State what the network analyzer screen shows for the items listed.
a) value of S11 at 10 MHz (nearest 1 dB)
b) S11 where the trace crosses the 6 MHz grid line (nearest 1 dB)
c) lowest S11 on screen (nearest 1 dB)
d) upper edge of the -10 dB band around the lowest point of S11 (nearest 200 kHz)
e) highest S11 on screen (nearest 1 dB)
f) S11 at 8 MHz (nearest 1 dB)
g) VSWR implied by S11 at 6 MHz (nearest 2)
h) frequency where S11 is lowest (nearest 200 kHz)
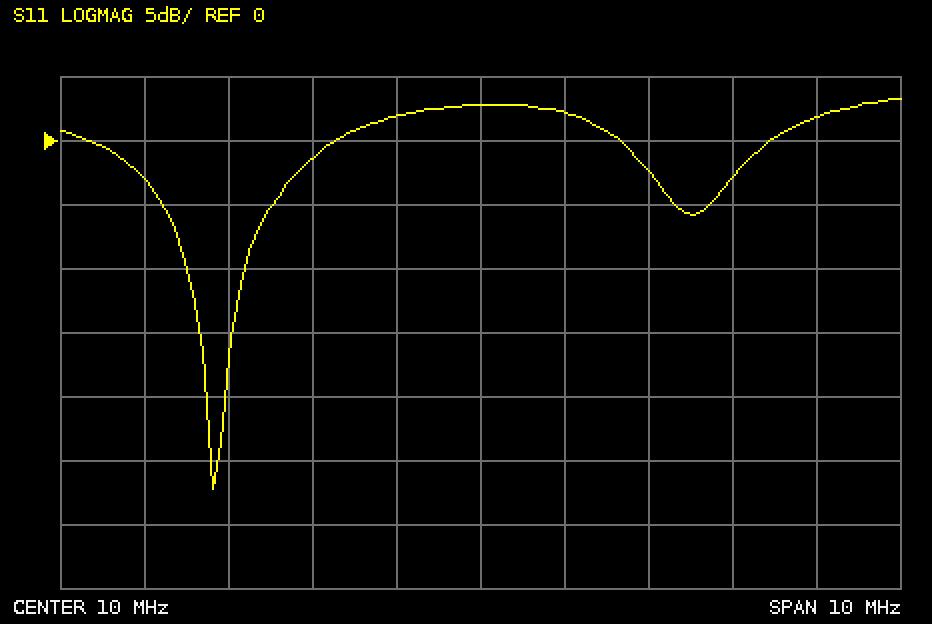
3 dB
-3 dB
-27 dB
7.2 MHz
3 dB
-1 dB
6
6.8 MHz
